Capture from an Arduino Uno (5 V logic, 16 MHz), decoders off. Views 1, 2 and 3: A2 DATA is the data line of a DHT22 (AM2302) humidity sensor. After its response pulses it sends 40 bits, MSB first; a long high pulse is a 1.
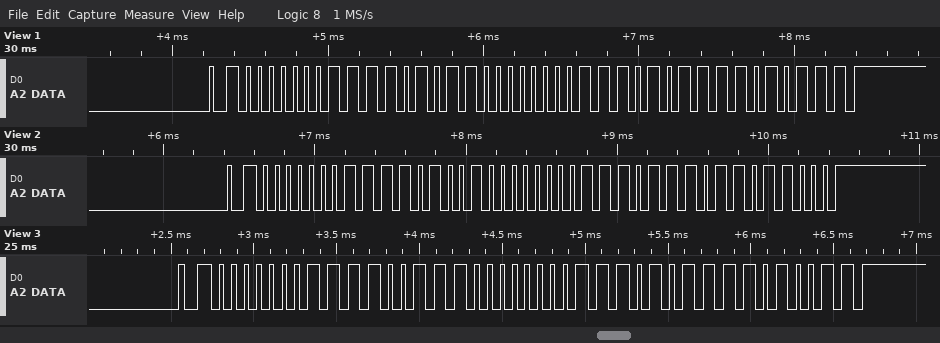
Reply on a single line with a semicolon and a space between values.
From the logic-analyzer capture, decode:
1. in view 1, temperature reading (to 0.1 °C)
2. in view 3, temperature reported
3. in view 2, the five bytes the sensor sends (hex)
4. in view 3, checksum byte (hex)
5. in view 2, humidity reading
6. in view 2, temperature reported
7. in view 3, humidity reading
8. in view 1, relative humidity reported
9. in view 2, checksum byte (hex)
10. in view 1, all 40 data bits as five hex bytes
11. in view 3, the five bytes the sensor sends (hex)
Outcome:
23.5 °C; 23.5 °C; 01 E9 00 EE D8; 0xD3; 48.9 %; 23.8 °C; 48.7 %; 49.1 %; 0xD8; 01 EB 00 EB D7; 01 E7 00 EB D3
